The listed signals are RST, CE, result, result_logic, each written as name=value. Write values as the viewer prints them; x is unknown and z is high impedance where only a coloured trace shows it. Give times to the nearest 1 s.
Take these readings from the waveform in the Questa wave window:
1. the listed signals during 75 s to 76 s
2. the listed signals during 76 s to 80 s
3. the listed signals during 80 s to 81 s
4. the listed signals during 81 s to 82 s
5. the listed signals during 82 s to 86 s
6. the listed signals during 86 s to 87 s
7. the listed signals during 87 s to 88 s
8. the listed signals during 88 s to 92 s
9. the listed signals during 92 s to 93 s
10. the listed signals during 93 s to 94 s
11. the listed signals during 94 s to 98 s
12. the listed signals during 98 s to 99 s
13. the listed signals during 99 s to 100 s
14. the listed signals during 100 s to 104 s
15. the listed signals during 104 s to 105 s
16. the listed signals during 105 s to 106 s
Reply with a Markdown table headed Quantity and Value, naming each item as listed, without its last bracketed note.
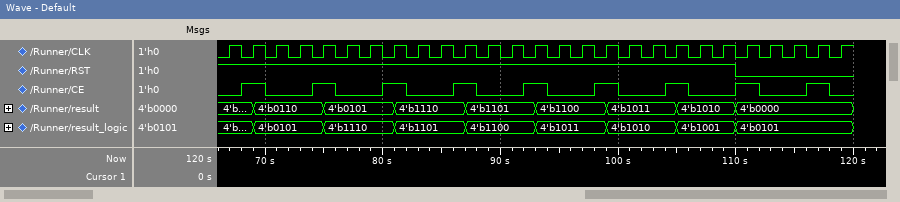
| Quantity | Value |
|---|---|
| the listed signals during 75 s to 76 s | RST=1, CE=1, result=4'b0101, result_logic=4'b1110 |
| the listed signals during 76 s to 80 s | RST=1, CE=0, result=4'b0101, result_logic=4'b1110 |
| the listed signals during 80 s to 81 s | RST=1, CE=1, result=4'b0101, result_logic=4'b1110 |
| the listed signals during 81 s to 82 s | RST=1, CE=1, result=4'b1110, result_logic=4'b1101 |
| the listed signals during 82 s to 86 s | RST=1, CE=0, result=4'b1110, result_logic=4'b1101 |
| the listed signals during 86 s to 87 s | RST=1, CE=1, result=4'b1110, result_logic=4'b1101 |
| the listed signals during 87 s to 88 s | RST=1, CE=1, result=4'b1101, result_logic=4'b1100 |
| the listed signals during 88 s to 92 s | RST=1, CE=0, result=4'b1101, result_logic=4'b1100 |
| the listed signals during 92 s to 93 s | RST=1, CE=1, result=4'b1101, result_logic=4'b1100 |
| the listed signals during 93 s to 94 s | RST=1, CE=1, result=4'b1100, result_logic=4'b1011 |
| the listed signals during 94 s to 98 s | RST=1, CE=0, result=4'b1100, result_logic=4'b1011 |
| the listed signals during 98 s to 99 s | RST=1, CE=1, result=4'b1100, result_logic=4'b1011 |
| the listed signals during 99 s to 100 s | RST=1, CE=1, result=4'b1011, result_logic=4'b1010 |
| the listed signals during 100 s to 104 s | RST=1, CE=0, result=4'b1011, result_logic=4'b1010 |
| the listed signals during 104 s to 105 s | RST=1, CE=1, result=4'b1011, result_logic=4'b1010 |
| the listed signals during 105 s to 106 s | RST=1, CE=1, result=4'b1010, result_logic=4'b1001 |
